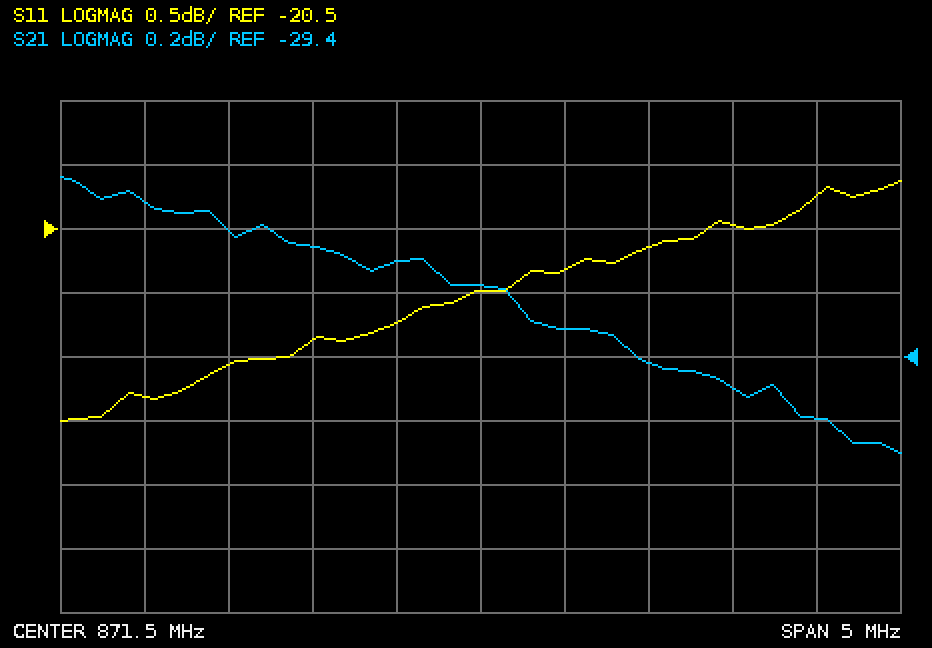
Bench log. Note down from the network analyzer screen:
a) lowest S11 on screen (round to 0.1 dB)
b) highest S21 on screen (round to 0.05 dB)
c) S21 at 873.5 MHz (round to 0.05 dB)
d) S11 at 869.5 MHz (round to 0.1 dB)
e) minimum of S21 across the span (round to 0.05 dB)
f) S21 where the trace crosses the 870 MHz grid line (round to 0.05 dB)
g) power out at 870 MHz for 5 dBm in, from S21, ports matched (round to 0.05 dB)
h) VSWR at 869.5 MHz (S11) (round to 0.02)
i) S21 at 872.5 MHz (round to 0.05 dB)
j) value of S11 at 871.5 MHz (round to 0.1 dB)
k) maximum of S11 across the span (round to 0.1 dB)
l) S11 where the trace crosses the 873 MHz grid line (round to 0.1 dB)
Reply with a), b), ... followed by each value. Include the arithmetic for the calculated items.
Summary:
a) -22.0 dB
b) -28.85 dB
c) -29.60 dB
d) -21.8 dB
e) -29.70 dB
f) -29.00 dB
g) 5 dBm + (-29.00 dB) = -24.00 dBm
h) |Γ| = 10^(-21.8/20) = 0.0813; VSWR = (1 + 0.0813)/(1 − 0.0813) ≈ 1.18
i) -29.40 dB
j) -21.0 dB
k) -20.1 dB
l) -20.5 dB
